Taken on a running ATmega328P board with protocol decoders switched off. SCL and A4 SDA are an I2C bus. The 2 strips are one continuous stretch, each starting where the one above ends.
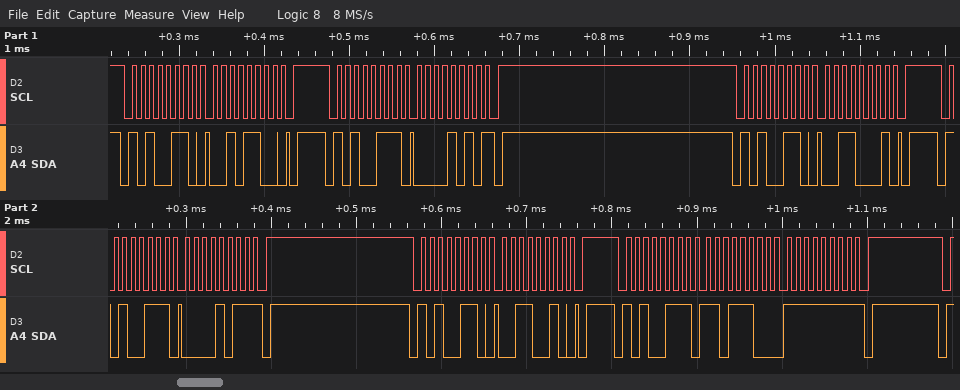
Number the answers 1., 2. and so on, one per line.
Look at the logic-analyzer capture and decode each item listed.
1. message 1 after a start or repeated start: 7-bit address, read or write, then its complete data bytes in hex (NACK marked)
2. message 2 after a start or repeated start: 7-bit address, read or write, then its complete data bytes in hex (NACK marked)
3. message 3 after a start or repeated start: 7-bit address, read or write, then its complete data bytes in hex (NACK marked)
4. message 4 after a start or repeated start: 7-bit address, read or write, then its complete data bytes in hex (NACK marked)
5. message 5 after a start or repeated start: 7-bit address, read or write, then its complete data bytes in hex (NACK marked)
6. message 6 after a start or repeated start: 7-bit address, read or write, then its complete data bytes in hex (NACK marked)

1. 0x53 write: 2C
2. 0x53 read: 0A NACK
3. 0x53 write: 31
4. 0x53 read: 0B NACK
5. 0x53 write: 32
6. 0x53 read: DC FF NACK
